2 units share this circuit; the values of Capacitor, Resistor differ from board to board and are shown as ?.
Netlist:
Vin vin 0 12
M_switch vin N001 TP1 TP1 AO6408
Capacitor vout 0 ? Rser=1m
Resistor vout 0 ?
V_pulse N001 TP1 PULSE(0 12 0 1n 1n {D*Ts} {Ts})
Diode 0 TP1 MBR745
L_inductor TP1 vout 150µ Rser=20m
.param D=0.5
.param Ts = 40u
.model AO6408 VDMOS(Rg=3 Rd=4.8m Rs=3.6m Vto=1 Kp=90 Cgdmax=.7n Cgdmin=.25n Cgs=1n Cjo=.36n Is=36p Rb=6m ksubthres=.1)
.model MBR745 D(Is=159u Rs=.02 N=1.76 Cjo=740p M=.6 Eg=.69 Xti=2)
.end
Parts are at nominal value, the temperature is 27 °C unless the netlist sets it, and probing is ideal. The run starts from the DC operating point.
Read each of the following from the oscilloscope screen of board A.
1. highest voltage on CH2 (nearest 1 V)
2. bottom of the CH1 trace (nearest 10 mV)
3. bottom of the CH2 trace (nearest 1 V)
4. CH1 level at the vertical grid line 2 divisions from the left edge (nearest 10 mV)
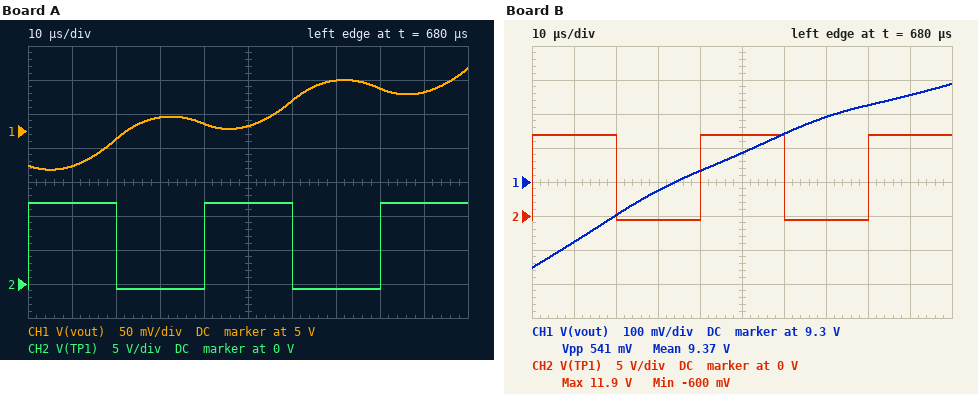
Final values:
12 V
4.94 V
-1 V
4.99 V
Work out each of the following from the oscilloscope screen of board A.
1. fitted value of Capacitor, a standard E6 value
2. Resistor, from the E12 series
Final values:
100 µF
0.47 Ω
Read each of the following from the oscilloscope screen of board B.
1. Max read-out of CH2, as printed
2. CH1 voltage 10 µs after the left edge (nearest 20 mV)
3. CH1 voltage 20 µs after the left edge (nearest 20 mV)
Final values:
11.9 V
9.12 V
9.20 V
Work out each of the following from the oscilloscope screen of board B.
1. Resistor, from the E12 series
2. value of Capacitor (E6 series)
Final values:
3.3 Ω
470 µF
